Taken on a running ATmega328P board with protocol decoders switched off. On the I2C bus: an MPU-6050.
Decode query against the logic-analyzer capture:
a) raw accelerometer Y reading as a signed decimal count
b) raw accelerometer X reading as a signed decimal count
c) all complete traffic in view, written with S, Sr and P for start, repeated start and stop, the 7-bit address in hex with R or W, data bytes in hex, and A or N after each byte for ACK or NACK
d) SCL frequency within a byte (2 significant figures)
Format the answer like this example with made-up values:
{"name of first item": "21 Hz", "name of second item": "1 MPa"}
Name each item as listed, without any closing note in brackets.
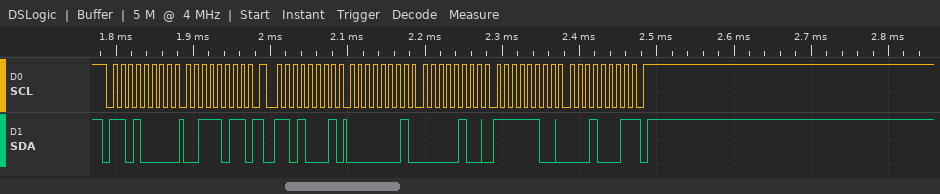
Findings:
{"raw accelerometer Y reading as a signed decimal count": "-1007", "raw accelerometer X reading as a signed decimal count": "260", "all complete traffic in view, written with S, Sr and P for start, repeated start and stop, the 7-bit address in hex with R or W, data bytes in hex, and A or N after each byte for ACK or NACK": "S 68W A 3B A Sr 68R A 01 A 04 A FC A 11 N P", "SCL frequency within a byte": "100 kHz"}
